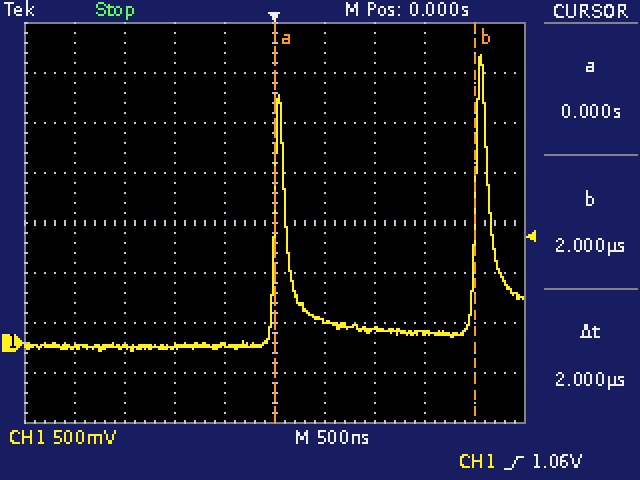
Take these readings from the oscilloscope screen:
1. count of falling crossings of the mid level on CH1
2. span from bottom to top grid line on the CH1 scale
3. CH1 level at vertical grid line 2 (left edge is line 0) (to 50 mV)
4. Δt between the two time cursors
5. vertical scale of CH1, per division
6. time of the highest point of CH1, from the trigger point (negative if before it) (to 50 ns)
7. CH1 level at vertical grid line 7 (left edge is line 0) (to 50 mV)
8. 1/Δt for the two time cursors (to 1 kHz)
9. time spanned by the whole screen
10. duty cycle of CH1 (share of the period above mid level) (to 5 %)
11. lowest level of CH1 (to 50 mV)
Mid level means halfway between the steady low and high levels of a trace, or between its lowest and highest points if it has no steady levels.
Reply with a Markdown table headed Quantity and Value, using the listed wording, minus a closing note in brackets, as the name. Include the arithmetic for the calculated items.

| Quantity | Value |
|---|---|
| count of falling crossings of the mid level on CH1 | 2 |
| span from bottom to top grid line on the CH1 scale | 4 V |
| CH1 level at vertical grid line 2 (left edge is line 0) | -50 mV |
| Δt between the two time cursors | 2 µs |
| vertical scale of CH1, per division | 500 mV |
| time of the highest point of CH1, from the trigger point (negative if before it) | +2.05 µs |
| CH1 level at vertical grid line 7 (left edge is line 0) | 150 mV |
| 1/Δt for the two time cursors | 1 / 2 µs ≈ 500 kHz |
| time spanned by the whole screen | 5 µs |
| duty cycle of CH1 (share of the period above mid level) | 5 % |
| lowest level of CH1 | -100 mV |
